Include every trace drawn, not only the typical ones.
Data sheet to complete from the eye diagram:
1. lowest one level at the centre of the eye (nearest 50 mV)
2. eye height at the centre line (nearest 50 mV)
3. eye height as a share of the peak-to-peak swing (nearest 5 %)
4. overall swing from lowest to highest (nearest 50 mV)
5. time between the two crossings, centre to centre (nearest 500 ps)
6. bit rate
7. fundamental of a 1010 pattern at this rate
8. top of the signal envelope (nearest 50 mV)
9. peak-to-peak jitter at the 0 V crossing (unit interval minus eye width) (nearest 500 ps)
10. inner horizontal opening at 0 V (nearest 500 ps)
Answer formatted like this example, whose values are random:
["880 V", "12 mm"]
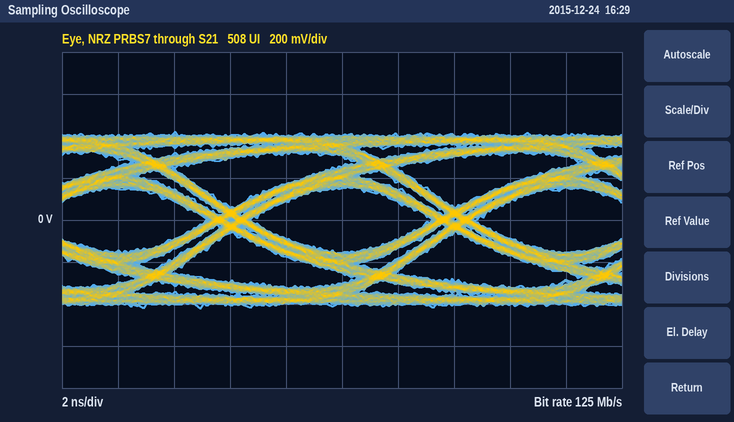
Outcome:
["150 mV", "300 mV", "35 %", "850 mV", "8.0 ns", "125 Mb/s", "62.5 MHz", "400 mV", "1.5 ns", "6.5 ns"]
